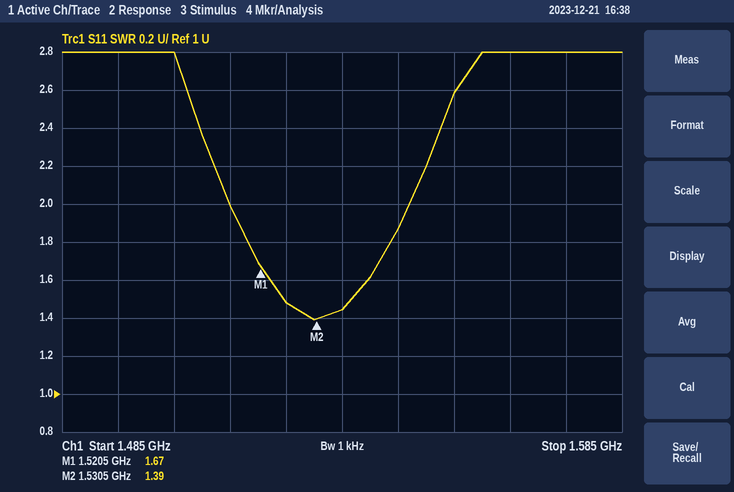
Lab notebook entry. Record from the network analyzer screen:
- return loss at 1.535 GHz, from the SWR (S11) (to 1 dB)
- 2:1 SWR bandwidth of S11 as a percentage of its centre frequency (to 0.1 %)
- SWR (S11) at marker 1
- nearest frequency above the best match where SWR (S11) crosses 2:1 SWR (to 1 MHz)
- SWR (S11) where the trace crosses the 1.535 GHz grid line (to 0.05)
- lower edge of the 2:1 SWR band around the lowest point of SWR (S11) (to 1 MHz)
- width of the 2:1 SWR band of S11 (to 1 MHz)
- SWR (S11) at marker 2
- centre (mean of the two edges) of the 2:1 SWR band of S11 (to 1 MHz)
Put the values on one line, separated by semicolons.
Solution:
15 dB; 2.1 %; 1.67; 1.547 GHz; 1.45; 1.515 GHz; 32 MHz; 1.39; 1.531 GHz
